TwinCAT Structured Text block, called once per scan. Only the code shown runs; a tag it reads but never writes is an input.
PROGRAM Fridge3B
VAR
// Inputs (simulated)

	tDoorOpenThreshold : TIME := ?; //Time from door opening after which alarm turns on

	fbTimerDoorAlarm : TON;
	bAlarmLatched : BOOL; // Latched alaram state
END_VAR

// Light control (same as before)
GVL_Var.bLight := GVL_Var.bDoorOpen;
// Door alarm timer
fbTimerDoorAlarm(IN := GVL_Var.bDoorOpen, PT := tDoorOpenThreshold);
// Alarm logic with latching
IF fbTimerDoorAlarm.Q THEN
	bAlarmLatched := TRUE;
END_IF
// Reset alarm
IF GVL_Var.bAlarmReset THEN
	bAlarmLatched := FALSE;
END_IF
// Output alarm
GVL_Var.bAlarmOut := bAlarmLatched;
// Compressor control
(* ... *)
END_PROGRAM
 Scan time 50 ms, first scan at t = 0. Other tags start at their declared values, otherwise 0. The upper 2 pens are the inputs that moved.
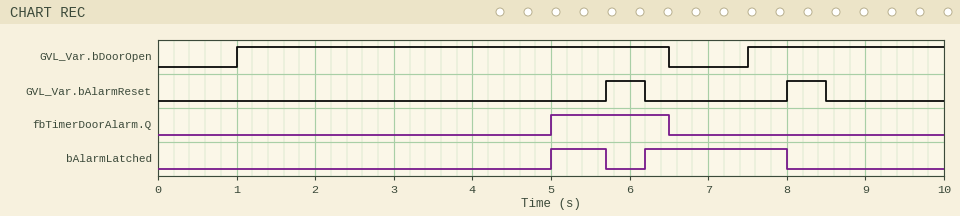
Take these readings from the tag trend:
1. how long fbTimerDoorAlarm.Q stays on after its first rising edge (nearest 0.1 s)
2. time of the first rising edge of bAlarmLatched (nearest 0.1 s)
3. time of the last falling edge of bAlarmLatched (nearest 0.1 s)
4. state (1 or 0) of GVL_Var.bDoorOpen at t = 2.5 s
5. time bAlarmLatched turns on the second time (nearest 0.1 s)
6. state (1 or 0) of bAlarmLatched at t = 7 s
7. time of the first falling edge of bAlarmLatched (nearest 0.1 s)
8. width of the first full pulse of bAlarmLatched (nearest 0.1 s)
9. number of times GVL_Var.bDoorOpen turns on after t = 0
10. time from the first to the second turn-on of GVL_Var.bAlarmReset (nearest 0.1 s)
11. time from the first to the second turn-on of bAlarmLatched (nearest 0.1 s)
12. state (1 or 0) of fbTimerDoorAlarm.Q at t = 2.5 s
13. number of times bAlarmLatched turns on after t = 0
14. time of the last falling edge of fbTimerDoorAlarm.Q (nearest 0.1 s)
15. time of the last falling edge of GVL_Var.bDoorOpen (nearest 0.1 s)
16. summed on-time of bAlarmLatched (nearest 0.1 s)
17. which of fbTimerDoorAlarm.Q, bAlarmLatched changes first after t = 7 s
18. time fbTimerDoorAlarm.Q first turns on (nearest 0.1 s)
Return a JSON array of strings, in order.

["1.5 s", "5.0 s", "8.0 s", "1", "6.2 s", "1", "5.7 s", "0.7 s", "2", "2.3 s", "1.2 s", "0", "2", "6.5 s", "6.5 s", "2.5 s", "bAlarmLatched", "5.0 s"]
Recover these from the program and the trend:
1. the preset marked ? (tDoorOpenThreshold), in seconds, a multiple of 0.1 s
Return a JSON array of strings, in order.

["4.0 s"]
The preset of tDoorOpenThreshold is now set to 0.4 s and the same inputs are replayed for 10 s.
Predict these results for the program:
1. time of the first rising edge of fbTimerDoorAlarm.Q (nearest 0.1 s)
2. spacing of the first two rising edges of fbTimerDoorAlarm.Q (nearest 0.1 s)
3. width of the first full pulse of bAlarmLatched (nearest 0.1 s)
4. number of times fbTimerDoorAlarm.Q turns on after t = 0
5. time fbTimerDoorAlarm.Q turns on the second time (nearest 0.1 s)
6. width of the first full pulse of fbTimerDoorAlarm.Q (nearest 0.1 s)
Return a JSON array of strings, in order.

["1.4 s", "6.5 s", "4.3 s", "2", "7.9 s", "5.1 s"]
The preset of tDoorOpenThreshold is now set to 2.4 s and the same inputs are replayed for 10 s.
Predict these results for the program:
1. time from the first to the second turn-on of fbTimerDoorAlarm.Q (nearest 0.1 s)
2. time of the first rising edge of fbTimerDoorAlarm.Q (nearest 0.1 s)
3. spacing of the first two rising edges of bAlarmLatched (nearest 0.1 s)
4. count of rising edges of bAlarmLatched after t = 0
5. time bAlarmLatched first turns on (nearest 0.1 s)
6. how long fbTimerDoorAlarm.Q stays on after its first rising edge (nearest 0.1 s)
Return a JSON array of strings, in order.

["6.5 s", "3.4 s", "2.8 s", "3", "3.4 s", "3.1 s"]
